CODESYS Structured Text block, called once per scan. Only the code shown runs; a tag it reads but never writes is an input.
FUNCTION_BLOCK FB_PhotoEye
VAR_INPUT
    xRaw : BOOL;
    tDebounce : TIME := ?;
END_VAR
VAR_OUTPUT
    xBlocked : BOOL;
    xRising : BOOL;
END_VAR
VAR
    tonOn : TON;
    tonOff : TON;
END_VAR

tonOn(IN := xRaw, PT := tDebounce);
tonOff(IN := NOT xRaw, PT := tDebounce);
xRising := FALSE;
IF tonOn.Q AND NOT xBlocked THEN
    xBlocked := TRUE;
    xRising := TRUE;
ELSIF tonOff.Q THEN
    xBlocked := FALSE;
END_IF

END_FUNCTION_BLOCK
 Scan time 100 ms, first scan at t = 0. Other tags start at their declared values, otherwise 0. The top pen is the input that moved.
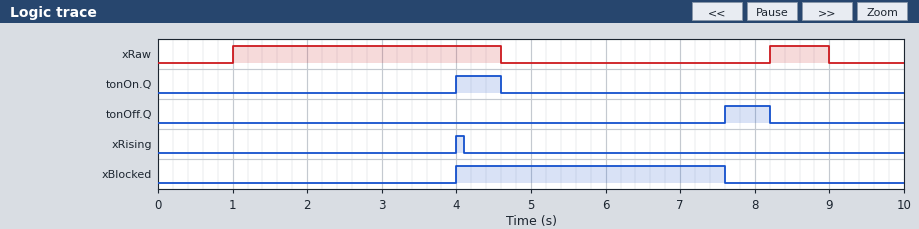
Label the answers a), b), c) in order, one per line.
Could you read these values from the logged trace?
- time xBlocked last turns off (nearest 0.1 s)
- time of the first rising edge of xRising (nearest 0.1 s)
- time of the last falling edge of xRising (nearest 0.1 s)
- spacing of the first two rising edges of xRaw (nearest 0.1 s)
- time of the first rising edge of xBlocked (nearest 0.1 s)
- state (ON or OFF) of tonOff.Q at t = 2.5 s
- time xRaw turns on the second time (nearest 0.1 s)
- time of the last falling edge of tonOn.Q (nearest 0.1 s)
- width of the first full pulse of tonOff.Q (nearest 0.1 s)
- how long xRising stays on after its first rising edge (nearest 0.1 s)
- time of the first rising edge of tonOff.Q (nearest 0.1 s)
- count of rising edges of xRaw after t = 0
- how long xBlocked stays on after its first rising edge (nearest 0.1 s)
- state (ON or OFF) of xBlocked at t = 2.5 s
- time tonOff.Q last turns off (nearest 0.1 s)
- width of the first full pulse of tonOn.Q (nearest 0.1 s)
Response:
a) 7.6 s
b) 4.0 s
c) 4.1 s
d) 7.2 s
e) 4.0 s
f) OFF
g) 8.2 s
h) 4.6 s
i) 0.6 s
j) 0.1 s
k) 7.6 s
l) 2
m) 3.6 s
n) OFF
o) 8.2 s
p) 0.6 s
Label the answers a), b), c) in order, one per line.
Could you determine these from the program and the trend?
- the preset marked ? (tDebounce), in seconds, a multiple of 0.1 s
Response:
a) 3.0 s
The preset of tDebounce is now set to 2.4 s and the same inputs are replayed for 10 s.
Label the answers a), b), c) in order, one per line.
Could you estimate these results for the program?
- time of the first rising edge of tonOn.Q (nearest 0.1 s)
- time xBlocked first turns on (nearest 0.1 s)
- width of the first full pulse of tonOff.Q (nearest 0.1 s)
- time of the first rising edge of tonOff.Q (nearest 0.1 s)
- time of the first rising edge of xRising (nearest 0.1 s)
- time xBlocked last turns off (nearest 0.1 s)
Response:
a) 3.4 s
b) 3.4 s
c) 1.2 s
d) 7.0 s
e) 3.4 s
f) 7.0 s
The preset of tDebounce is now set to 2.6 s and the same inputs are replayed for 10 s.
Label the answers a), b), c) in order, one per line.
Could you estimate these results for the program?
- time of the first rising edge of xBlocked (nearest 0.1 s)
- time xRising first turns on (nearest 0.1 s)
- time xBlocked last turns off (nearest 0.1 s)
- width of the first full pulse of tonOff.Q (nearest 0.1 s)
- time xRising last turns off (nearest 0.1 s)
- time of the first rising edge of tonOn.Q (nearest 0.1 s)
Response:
a) 3.6 s
b) 3.6 s
c) 7.2 s
d) 1.0 s
e) 3.7 s
f) 3.6 s
